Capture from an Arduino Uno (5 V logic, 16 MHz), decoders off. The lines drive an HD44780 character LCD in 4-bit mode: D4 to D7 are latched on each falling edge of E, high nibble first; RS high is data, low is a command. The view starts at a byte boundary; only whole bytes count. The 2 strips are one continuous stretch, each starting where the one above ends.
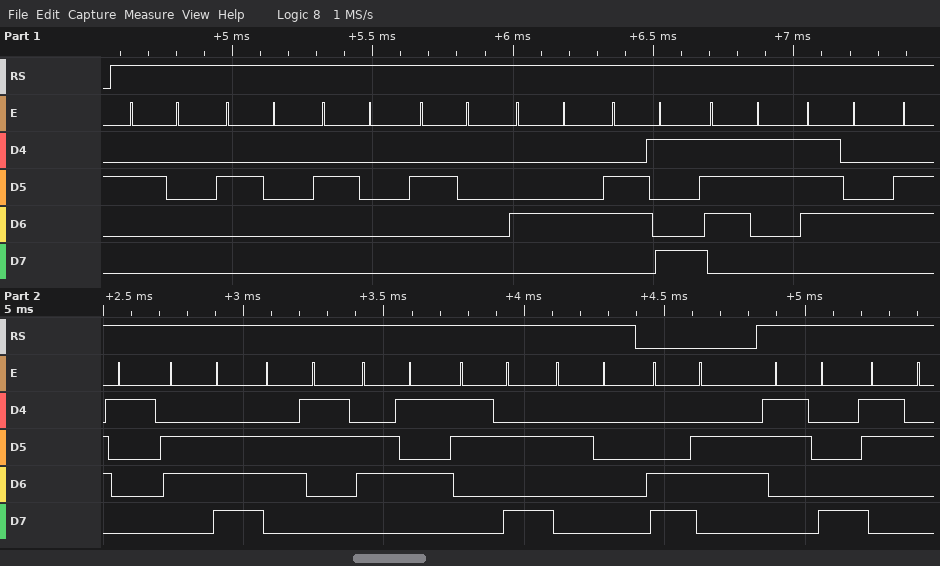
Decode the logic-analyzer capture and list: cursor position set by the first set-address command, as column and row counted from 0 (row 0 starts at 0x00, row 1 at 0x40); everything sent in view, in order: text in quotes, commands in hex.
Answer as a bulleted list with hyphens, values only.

- column 6, row 1
- "    Distance: " 0xC6 "82"
